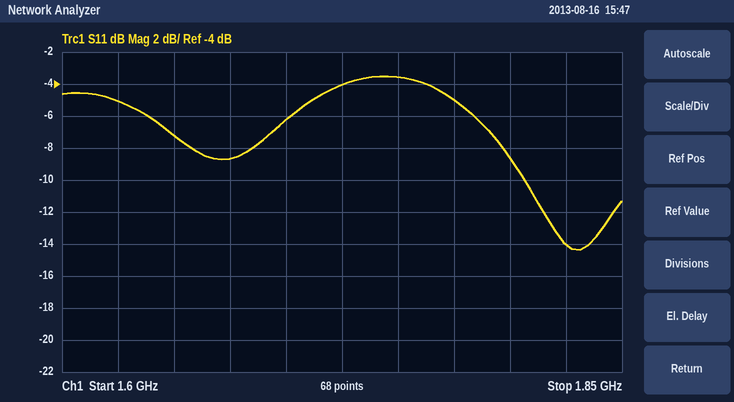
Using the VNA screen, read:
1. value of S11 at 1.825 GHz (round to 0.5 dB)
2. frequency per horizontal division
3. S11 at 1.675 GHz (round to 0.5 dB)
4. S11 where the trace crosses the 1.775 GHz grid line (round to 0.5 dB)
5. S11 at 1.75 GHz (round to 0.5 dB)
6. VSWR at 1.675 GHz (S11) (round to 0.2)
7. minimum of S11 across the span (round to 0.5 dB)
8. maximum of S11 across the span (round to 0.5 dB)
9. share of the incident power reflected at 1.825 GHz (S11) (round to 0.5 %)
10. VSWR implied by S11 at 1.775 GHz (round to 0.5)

-14.0 dB
25 MHz
-8.5 dB
-5.0 dB
-3.5 dB
2.2
-14.5 dB
-3.5 dB
4.0 %
3.5
